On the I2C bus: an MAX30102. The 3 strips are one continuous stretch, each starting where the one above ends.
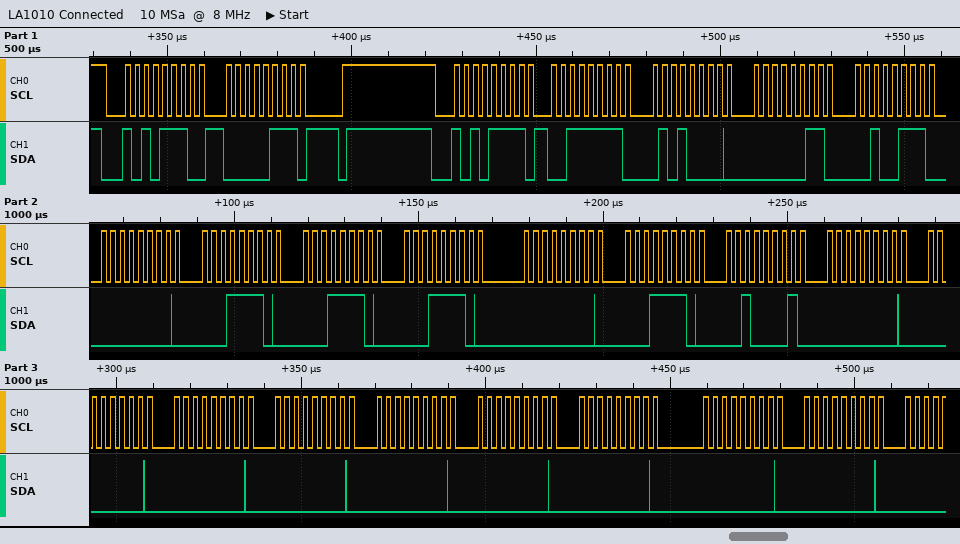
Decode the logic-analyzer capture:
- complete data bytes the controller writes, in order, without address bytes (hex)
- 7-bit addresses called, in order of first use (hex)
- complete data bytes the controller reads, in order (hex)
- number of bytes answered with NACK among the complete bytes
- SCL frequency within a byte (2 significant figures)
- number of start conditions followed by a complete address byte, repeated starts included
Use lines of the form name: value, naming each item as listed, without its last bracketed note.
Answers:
complete data bytes the controller writes, in order, without address bytes: 07
7-bit addresses called, in order of first use: 0x57
complete data bytes the controller reads, in order: 3F 50 03 27 00 1E 1E 1E 00 1E 21 00 00 00 00 00 00 00 00 00
number of bytes answered with NACK among the complete bytes: 0
SCL frequency within a byte: 400 kHz
number of start conditions followed by a complete address byte, repeated starts included: 2
